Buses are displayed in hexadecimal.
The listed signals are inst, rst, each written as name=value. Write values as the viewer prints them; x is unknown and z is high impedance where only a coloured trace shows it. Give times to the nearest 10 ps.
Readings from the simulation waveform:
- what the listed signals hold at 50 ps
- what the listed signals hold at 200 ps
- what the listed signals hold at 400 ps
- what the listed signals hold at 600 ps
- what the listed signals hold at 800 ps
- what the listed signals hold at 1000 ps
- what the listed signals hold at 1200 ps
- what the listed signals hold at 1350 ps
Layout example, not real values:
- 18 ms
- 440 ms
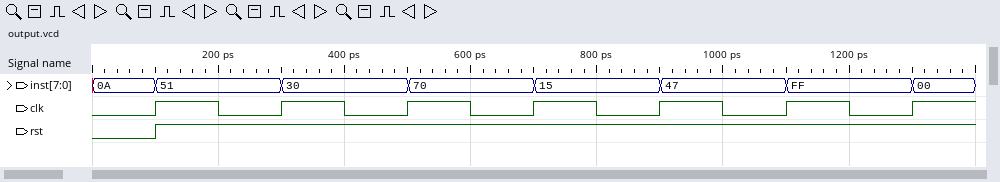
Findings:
- inst=0A, rst=0
- inst=51, rst=1
- inst=30, rst=1
- inst=70, rst=1
- inst=15, rst=1
- inst=47, rst=1
- inst=FF, rst=1
- inst=00, rst=1
